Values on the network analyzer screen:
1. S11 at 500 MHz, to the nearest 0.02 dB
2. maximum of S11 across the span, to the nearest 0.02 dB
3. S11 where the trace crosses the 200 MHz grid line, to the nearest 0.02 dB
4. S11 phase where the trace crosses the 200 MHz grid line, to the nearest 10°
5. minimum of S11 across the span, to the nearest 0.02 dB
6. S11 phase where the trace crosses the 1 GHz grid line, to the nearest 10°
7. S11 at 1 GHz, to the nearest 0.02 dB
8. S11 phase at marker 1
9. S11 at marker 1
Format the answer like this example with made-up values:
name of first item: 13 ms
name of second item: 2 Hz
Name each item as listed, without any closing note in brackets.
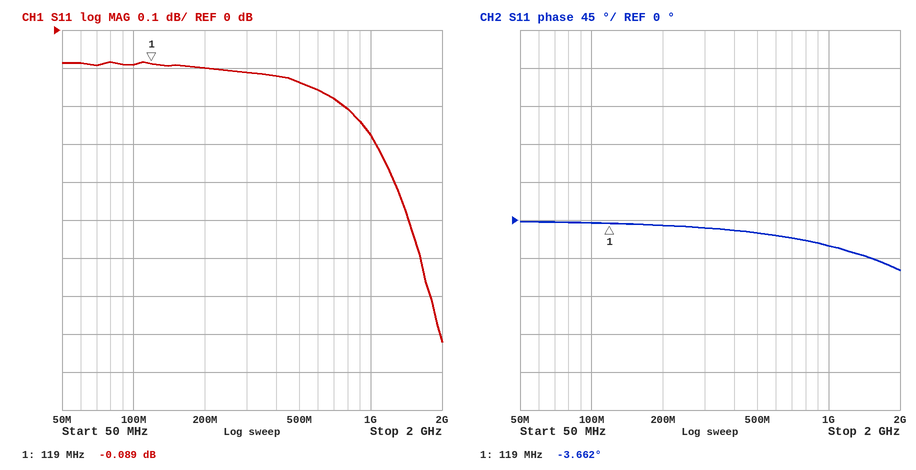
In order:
S11 at 500 MHz, to the nearest 0.02 dB: -0.14 dB
maximum of S11 across the span, to the nearest 0.02 dB: -0.08 dB
S11 where the trace crosses the 200 MHz grid line, to the nearest 0.02 dB: -0.10 dB
S11 phase where the trace crosses the 200 MHz grid line, to the nearest 10°: -10°
minimum of S11 across the span, to the nearest 0.02 dB: -0.82 dB
S11 phase where the trace crosses the 1 GHz grid line, to the nearest 10°: -30°
S11 at 1 GHz, to the nearest 0.02 dB: -0.28 dB
S11 phase at marker 1: -3.662°
S11 at marker 1: -0.089 dB
